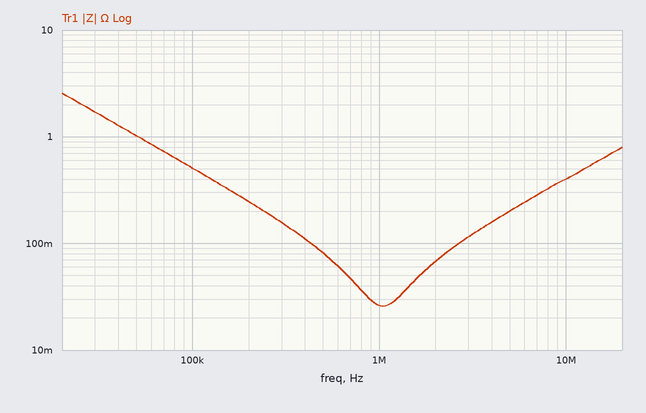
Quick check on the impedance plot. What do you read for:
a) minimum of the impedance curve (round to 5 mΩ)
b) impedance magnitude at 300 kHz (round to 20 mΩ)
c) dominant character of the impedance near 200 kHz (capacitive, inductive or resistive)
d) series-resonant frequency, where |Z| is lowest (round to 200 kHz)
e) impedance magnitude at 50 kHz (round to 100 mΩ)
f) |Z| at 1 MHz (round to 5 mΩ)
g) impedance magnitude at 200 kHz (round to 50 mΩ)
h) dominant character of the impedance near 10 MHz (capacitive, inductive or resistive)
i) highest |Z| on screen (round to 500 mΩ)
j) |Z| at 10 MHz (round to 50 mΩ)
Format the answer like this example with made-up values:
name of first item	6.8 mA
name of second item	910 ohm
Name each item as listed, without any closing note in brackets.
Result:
minimum of the impedance curve	25 mΩ
impedance magnitude at 300 kHz	160 mΩ
dominant character of the impedance near 200 kHz	capacitive
series-resonant frequency, where |Z| is lowest	1.0 MHz
impedance magnitude at 50 kHz	1.0 Ω
|Z| at 1 MHz	25 mΩ
impedance magnitude at 200 kHz	250 mΩ
dominant character of the impedance near 10 MHz	inductive
highest |Z| on screen	2.5 Ω
|Z| at 10 MHz	400 mΩ
